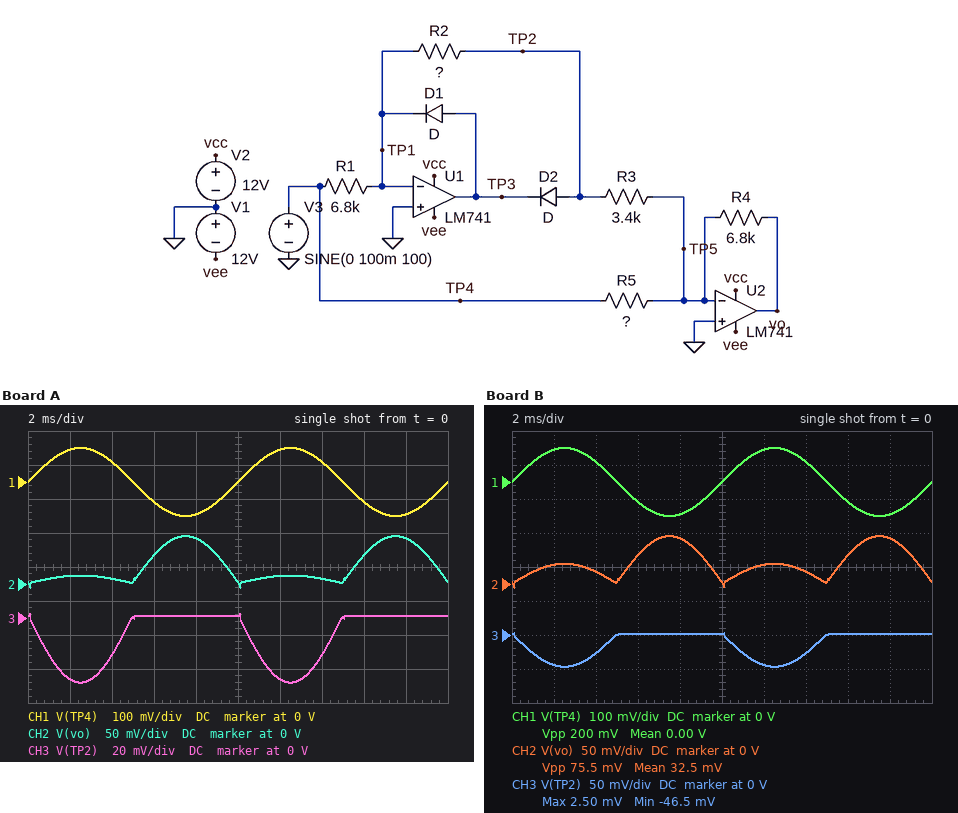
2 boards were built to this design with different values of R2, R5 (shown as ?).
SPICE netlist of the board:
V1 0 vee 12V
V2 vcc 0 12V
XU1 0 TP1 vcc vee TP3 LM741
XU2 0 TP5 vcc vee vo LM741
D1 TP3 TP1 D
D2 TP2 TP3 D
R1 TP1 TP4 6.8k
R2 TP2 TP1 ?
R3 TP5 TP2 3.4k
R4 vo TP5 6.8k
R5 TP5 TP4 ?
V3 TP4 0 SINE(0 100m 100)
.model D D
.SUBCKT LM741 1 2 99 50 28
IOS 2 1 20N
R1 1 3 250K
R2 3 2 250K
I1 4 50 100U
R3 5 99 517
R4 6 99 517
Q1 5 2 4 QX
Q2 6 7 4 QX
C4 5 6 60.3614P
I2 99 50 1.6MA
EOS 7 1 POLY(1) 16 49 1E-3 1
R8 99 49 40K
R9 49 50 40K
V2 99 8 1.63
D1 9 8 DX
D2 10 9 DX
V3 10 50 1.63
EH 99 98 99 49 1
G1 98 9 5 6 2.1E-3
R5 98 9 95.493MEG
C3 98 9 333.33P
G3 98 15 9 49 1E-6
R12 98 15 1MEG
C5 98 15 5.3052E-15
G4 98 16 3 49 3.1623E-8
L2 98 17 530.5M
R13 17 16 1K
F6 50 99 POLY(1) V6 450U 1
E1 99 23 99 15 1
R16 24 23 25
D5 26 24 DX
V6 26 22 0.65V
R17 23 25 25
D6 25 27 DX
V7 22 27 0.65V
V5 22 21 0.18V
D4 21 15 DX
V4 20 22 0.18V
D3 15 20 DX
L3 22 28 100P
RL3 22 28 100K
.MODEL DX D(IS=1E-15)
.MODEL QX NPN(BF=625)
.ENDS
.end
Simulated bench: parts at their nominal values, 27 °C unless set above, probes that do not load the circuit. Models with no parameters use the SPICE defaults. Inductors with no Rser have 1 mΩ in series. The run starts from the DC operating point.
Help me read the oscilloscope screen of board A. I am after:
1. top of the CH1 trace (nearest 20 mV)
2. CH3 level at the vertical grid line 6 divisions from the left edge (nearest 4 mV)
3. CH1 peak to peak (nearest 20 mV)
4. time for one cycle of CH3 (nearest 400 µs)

100 mV
-36 mV
200 mV
10.0 ms
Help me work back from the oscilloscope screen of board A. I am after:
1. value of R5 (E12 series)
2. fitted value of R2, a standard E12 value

10 kΩ
2.7 kΩ
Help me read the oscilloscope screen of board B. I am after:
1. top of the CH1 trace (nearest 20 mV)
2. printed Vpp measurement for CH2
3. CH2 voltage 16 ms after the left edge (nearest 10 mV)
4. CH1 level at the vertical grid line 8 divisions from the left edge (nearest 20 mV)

100 mV
75.5 mV
40 mV
-60 mV
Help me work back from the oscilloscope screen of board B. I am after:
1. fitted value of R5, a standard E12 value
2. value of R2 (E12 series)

10 kΩ
3.3 kΩ
